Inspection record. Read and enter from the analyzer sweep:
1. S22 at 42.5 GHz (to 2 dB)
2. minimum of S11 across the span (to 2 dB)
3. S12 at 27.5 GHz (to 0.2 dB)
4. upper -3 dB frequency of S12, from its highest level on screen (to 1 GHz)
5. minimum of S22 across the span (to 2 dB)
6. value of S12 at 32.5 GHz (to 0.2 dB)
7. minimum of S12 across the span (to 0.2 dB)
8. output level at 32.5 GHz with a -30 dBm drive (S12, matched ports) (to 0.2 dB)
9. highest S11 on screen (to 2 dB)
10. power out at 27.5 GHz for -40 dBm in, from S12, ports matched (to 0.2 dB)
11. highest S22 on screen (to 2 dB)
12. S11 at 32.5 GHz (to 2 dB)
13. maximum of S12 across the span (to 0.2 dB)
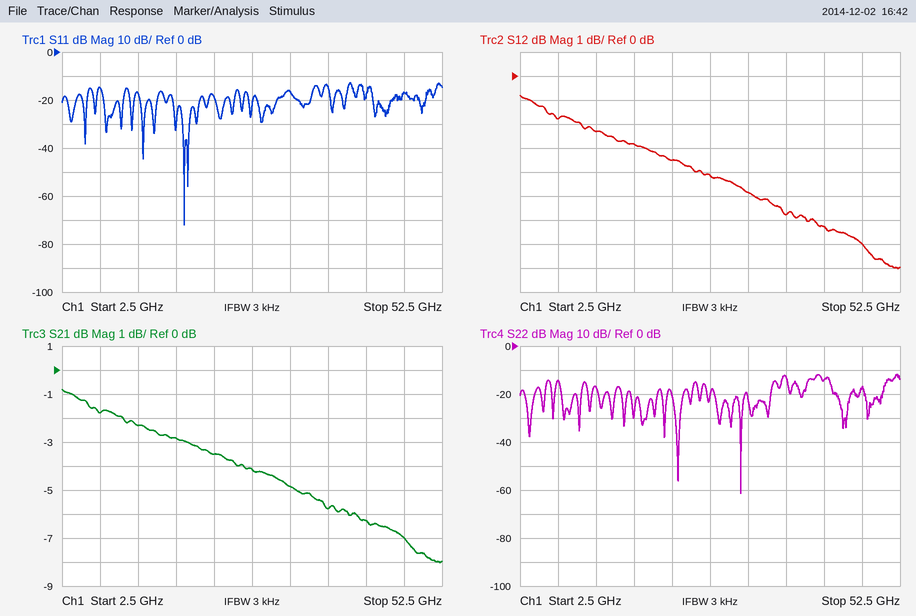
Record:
-14 dB
-72 dB
-4.2 dB
25 GHz
-62 dB
-4.8 dB
-8.0 dB
-34.8 dBm
-12 dB
-44.2 dBm
-12 dB
-16 dB
-0.8 dB
